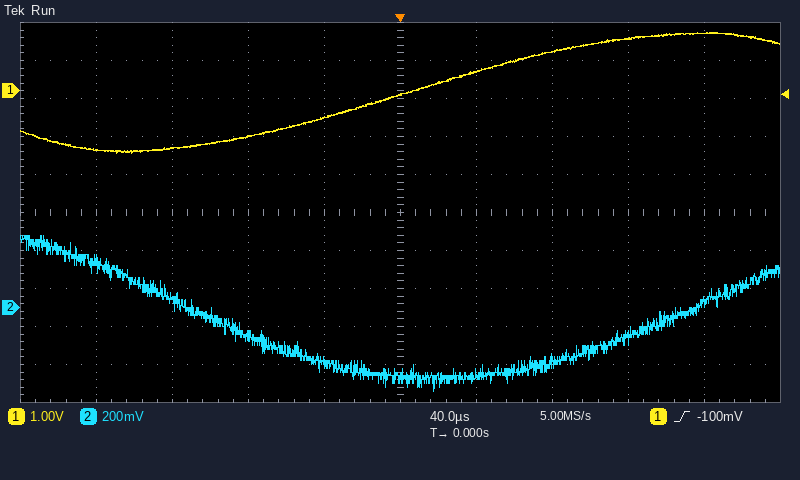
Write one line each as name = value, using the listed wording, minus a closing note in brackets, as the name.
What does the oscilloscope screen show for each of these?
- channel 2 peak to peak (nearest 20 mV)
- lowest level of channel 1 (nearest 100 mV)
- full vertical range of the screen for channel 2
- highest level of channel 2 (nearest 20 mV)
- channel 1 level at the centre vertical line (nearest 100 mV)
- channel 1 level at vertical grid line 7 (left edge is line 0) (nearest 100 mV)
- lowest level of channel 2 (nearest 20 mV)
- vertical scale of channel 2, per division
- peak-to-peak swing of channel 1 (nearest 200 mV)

channel 2 peak to peak = 820 mV
lowest level of channel 1 = -1.6 V
full vertical range of the screen for channel 2 = 2 V
highest level of channel 2 = 380 mV
channel 1 level at the centre vertical line = -100 mV
channel 1 level at vertical grid line 7 (left edge is line 0) = 1.0 V
lowest level of channel 2 = -440 mV
vertical scale of channel 2, per division = 200 mV
peak-to-peak swing of channel 1 = 3.2 V
